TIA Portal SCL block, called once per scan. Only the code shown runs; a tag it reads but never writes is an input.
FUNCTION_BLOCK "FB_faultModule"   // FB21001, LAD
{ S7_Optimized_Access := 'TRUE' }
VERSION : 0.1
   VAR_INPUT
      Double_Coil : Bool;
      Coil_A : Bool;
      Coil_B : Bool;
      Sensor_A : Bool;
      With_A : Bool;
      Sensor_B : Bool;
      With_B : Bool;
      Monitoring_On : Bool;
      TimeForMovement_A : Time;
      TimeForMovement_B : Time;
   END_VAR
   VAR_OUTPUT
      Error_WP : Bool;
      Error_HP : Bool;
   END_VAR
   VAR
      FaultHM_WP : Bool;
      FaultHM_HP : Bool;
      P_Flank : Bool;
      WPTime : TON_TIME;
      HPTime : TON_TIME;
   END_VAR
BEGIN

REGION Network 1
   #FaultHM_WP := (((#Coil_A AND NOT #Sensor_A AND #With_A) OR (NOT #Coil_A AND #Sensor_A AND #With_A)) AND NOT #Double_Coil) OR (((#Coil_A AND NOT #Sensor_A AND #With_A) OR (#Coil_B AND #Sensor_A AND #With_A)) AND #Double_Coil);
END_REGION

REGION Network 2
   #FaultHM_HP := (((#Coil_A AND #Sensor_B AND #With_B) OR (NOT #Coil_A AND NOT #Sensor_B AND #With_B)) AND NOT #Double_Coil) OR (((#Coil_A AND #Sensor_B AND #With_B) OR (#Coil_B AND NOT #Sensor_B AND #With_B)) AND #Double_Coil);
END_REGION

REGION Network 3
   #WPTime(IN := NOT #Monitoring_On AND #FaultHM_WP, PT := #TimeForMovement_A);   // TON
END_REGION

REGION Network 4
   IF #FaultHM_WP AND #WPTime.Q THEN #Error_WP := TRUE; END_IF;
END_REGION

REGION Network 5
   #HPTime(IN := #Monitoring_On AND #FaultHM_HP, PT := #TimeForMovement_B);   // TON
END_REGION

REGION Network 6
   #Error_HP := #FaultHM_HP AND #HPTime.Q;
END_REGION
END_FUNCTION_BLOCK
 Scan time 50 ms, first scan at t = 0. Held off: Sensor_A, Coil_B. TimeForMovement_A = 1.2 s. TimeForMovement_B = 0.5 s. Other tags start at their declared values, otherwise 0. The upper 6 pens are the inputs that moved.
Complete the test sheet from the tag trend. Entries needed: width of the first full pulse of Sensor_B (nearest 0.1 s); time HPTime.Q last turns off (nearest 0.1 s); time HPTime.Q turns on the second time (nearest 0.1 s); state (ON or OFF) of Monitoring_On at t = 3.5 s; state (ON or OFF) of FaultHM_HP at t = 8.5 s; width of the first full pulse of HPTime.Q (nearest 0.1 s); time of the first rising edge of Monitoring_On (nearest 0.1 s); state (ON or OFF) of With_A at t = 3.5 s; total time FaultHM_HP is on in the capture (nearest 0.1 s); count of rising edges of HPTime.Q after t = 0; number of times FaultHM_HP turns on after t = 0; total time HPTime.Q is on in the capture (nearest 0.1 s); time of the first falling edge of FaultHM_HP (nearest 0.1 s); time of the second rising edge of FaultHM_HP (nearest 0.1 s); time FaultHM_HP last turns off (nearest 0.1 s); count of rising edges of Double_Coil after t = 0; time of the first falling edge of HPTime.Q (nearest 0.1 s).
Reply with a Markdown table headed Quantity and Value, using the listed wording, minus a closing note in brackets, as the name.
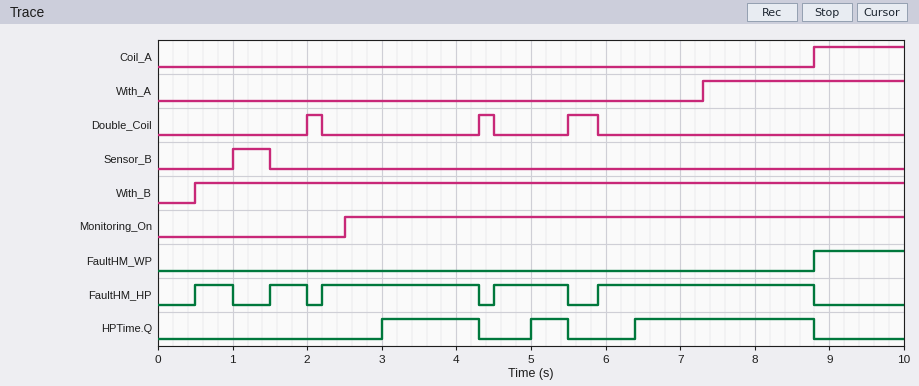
| Quantity | Value |
|---|---|
| width of the first full pulse of Sensor_B | 0.5 s |
| time HPTime.Q last turns off | 8.8 s |
| time HPTime.Q turns on the second time | 5.0 s |
| state (ON or OFF) of Monitoring_On at t = 3.5 s | ON |
| state (ON or OFF) of FaultHM_HP at t = 8.5 s | ON |
| width of the first full pulse of HPTime.Q | 1.3 s |
| time of the first rising edge of Monitoring_On | 2.5 s |
| state (ON or OFF) of With_A at t = 3.5 s | OFF |
| total time FaultHM_HP is on in the capture | 7.0 s |
| count of rising edges of HPTime.Q after t = 0 | 3 |
| number of times FaultHM_HP turns on after t = 0 | 5 |
| total time HPTime.Q is on in the capture | 4.2 s |
| time of the first falling edge of FaultHM_HP | 1.0 s |
| time of the second rising edge of FaultHM_HP | 1.5 s |
| time FaultHM_HP last turns off | 8.8 s |
| count of rising edges of Double_Coil after t = 0 | 3 |
| time of the first falling edge of HPTime.Q | 4.3 s |
